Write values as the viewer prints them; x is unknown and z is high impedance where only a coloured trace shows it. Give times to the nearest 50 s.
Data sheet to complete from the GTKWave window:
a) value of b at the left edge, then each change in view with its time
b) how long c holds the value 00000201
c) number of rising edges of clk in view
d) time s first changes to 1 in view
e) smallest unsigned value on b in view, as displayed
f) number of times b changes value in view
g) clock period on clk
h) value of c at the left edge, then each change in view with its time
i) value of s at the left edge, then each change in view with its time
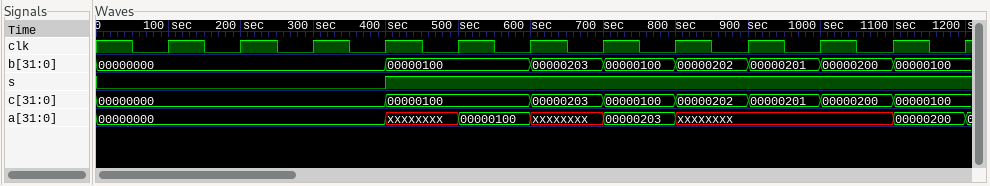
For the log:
00000000, 00000100 at 400 s, 00000203 at 600 s, 00000100 at 700 s, 00000202 at 800 s, 00000201 at 900 s, 00000200 at 1000 s, 00000100 at 1100 s
100 s
12
400 s
00000000
7
100 s
00000000, 00000100 at 400 s, 00000203 at 600 s, 00000100 at 700 s, 00000202 at 800 s, 00000201 at 900 s, 00000200 at 1000 s, 00000100 at 1100 s
0, 1 at 400 s
